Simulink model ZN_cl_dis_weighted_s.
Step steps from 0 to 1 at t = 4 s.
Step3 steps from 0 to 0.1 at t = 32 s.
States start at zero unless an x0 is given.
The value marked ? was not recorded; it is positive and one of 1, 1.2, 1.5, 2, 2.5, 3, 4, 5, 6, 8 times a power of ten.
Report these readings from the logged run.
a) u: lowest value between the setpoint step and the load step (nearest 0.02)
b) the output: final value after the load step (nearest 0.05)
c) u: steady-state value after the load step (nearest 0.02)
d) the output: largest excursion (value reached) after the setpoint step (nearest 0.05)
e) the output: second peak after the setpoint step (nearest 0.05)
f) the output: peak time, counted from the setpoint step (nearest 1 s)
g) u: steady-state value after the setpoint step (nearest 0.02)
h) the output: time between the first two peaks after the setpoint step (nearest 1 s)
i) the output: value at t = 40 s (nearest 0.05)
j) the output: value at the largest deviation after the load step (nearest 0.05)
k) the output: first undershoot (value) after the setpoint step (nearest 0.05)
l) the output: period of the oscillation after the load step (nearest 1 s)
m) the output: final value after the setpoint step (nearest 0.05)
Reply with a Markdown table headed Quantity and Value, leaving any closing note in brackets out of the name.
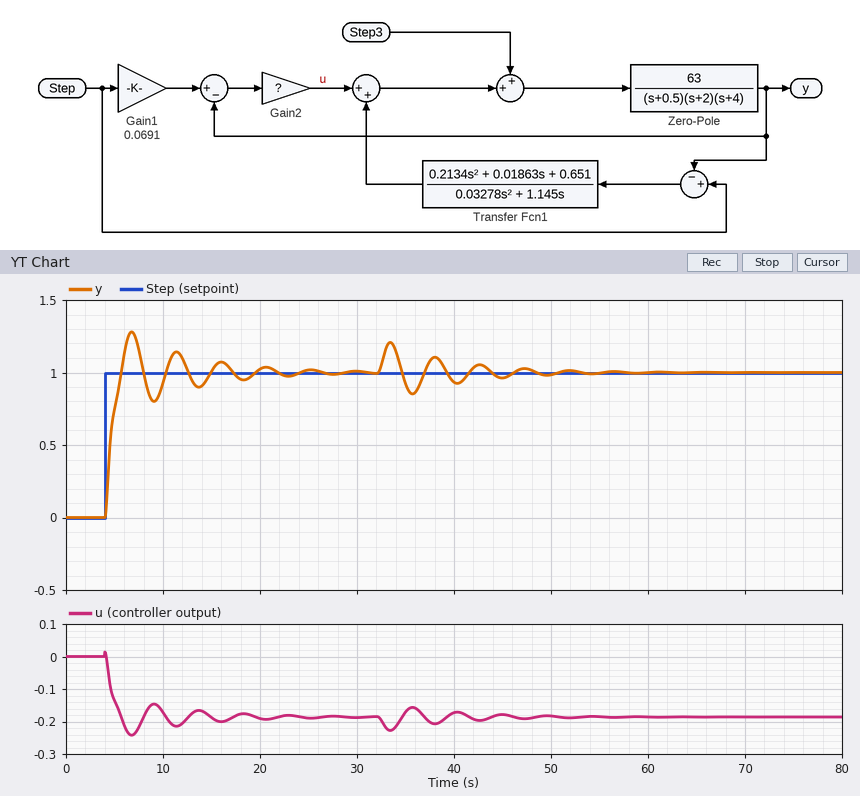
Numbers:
| Quantity | Value |
|---|---|
| u: lowest value between the setpoint step and the load step | -0.24 |
| the output: final value after the load step | 1.00 |
| u: steady-state value after the load step | -0.18 |
| the output: largest excursion (value reached) after the setpoint step | 1.30 |
| the output: second peak after the setpoint step | 1.15 |
| the output: peak time, counted from the setpoint step | 3 s |
| u: steady-state value after the setpoint step | -0.18 |
| the output: time between the first two peaks after the setpoint step | 5 s |
| the output: value at t = 40 s | 0.95 |
| the output: value at the largest deviation after the load step | 1.20 |
| the output: first undershoot (value) after the setpoint step | 0.80 |
| the output: period of the oscillation after the load step | 5 s |
| the output: final value after the setpoint step | 1.00 |
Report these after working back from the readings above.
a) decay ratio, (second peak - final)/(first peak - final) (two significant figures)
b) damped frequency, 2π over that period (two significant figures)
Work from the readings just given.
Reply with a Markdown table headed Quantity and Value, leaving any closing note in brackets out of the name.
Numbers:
| Quantity | Value |
|---|---|
| decay ratio, (second peak - final)/(first peak - final) | 0.50 |
| damped frequency, 2π over that period | 1.3 rad/s |
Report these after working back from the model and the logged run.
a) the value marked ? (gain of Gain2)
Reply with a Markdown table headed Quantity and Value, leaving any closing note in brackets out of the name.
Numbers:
| Quantity | Value |
|---|---|
| the value marked ? | 0.2 |
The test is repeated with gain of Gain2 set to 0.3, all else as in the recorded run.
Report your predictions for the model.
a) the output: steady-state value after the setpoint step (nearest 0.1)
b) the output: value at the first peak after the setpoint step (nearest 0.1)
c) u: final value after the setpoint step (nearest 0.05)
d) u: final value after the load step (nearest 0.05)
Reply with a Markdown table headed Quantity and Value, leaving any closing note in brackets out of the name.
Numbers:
| Quantity | Value |
|---|---|
| the output: steady-state value after the setpoint step | 1.0 |
| the output: value at the first peak after the setpoint step | 1.2 |
| u: final value after the setpoint step | -0.30 |
| u: final value after the load step | -0.30 |
